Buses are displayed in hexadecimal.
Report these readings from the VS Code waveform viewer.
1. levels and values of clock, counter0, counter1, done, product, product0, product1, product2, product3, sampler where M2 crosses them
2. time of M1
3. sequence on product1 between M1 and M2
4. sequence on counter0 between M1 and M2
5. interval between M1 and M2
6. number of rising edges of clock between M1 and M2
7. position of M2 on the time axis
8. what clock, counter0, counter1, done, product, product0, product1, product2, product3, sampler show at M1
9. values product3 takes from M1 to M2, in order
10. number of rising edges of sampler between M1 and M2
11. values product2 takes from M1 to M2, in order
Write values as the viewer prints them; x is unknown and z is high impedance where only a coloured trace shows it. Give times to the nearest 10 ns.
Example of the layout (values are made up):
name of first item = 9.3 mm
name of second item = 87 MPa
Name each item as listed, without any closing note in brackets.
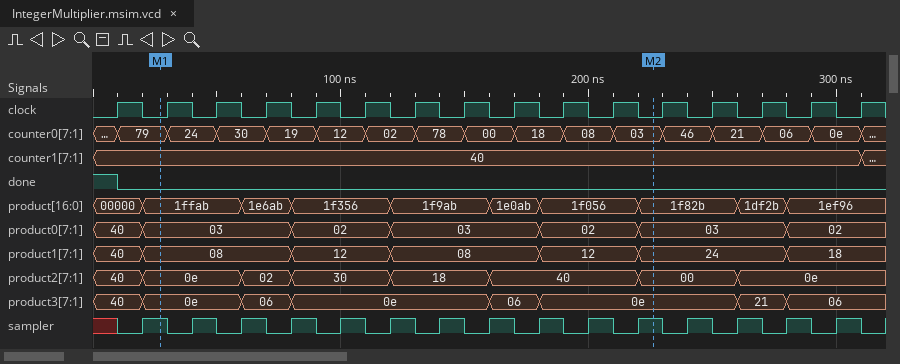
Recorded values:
levels and values of clock, counter0, counter1, done, product, product0, product1, product2, product3, sampler where M2 crosses them = clock=0, counter0=03, counter1=40, done=0, product=1f82b, product0=03, product1=24, product2=00, product3=0e, sampler=1
time of M1 = 30 ns
sequence on product1 between M1 and M2 = 08, 12, 08, 12, 24
sequence on counter0 between M1 and M2 = 79, 24, 30, 19, 12, 02, 78, 00, 18, 08, 03
interval between M1 and M2 = 200 ns
number of rising edges of clock between M1 and M2 = 10
position of M2 on the time axis = 230 ns
what clock, counter0, counter1, done, product, product0, product1, product2, product3, sampler show at M1 = clock=0, counter0=79, counter1=40, done=0, product=1ffab, product0=03, product1=08, product2=0e, product3=0e, sampler=1
values product3 takes from M1 to M2, in order = 0e, 06, 0e, 06, 0e
number of rising edges of sampler between M1 and M2 = 10
values product2 takes from M1 to M2, in order = 0e, 02, 30, 18, 40, 00
